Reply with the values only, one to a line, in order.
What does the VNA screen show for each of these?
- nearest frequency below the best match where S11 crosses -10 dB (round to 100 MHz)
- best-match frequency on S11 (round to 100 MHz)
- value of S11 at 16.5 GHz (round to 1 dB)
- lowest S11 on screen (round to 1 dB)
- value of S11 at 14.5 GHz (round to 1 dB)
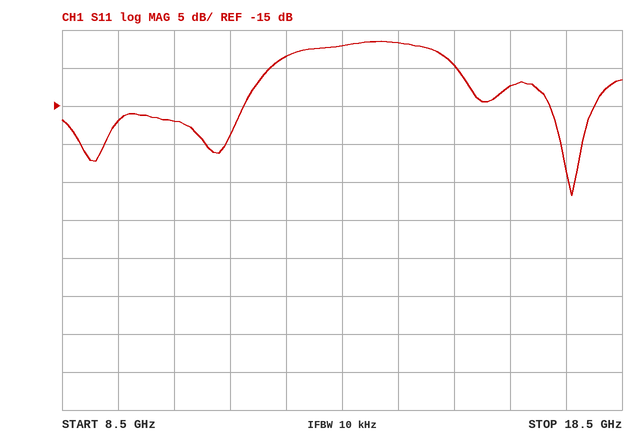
15.5 GHz
17.6 GHz
-12 dB
-27 dB
-7 dB
